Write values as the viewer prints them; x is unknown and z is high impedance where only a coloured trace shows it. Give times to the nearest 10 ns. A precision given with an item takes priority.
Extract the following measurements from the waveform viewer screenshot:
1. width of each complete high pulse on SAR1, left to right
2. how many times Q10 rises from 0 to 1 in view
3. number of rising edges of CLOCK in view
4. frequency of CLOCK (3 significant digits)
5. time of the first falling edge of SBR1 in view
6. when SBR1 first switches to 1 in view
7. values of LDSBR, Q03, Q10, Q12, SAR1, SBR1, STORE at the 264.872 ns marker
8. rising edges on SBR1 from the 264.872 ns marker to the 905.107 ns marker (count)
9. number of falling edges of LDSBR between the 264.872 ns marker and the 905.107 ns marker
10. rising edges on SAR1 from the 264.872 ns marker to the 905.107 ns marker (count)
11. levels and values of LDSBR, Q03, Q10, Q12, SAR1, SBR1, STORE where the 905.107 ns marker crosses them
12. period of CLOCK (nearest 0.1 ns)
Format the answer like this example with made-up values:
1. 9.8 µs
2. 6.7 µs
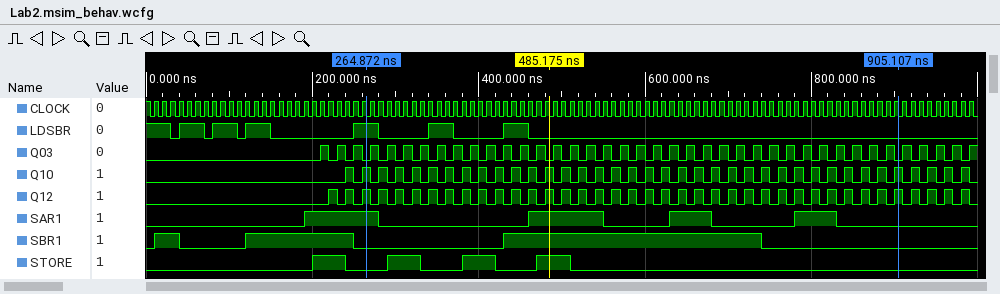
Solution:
1. 90 ns, 90 ns, 50 ns, 50 ns
2. 38
3. 99
4. 100 MHz
5. 40 ns
6. 10 ns
7. LDSBR=1, Q03=0, Q10=1, Q12=1, SAR1=1, SBR1=0, STORE=0
8. 1
9. 3
10. 3
11. LDSBR=0, Q03=0, Q10=1, Q12=1, SAR1=0, SBR1=0, STORE=0
12. 10 ns
